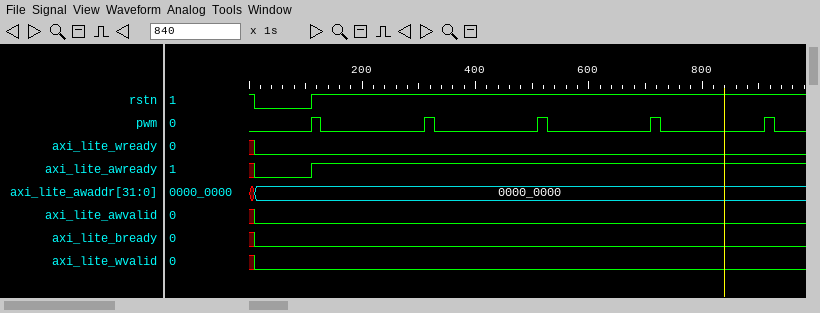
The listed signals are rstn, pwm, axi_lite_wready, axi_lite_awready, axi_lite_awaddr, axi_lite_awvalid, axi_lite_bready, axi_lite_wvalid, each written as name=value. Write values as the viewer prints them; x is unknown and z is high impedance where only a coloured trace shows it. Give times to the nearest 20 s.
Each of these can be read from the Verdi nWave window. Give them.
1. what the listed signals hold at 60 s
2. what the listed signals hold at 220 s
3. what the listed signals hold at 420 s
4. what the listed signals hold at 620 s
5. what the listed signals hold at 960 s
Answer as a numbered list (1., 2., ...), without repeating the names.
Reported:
1. rstn=0, pwm=0, axi_lite_wready=0, axi_lite_awready=0, axi_lite_awaddr=0000_0000, axi_lite_awvalid=0, axi_lite_bready=0, axi_lite_wvalid=0
2. rstn=1, pwm=0, axi_lite_wready=0, axi_lite_awready=1, axi_lite_awaddr=0000_0000, axi_lite_awvalid=0, axi_lite_bready=0, axi_lite_wvalid=0
3. rstn=1, pwm=0, axi_lite_wready=0, axi_lite_awready=1, axi_lite_awaddr=0000_0000, axi_lite_awvalid=0, axi_lite_bready=0, axi_lite_wvalid=0
4. rstn=1, pwm=0, axi_lite_wready=0, axi_lite_awready=1, axi_lite_awaddr=0000_0000, axi_lite_awvalid=0, axi_lite_bready=0, axi_lite_wvalid=0
5. rstn=1, pwm=0, axi_lite_wready=0, axi_lite_awready=1, axi_lite_awaddr=0000_0000, axi_lite_awvalid=0, axi_lite_bready=0, axi_lite_wvalid=0
